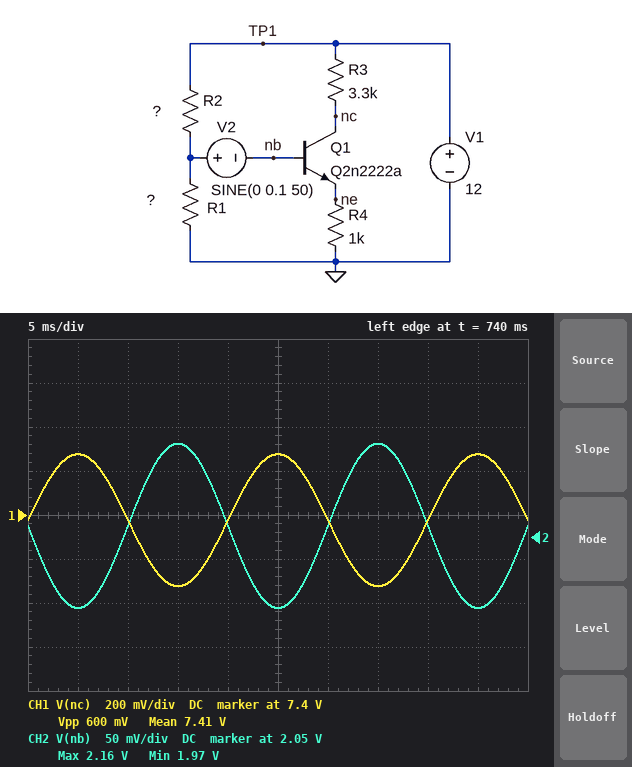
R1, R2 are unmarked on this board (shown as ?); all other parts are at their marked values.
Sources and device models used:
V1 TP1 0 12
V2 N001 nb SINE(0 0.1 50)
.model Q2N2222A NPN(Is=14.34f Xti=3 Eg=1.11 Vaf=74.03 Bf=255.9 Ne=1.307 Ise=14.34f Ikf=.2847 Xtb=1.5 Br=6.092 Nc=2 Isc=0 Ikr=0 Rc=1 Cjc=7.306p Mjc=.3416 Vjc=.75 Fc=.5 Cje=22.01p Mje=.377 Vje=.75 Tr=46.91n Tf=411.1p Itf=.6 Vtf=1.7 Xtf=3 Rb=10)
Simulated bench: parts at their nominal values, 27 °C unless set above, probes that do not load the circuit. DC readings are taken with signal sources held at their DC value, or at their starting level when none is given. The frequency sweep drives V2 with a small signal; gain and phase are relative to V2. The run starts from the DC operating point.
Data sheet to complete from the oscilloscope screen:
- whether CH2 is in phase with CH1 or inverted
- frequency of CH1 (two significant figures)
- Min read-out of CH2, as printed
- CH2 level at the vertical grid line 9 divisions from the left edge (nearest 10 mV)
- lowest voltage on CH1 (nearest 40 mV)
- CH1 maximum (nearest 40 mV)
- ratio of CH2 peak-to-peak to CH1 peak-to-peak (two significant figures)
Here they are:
inverted
50 Hz
1.97 V
1.97 V
7.08 V
7.68 V
0.31
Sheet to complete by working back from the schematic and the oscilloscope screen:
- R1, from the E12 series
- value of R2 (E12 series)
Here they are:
15 kΩ
68 kΩ
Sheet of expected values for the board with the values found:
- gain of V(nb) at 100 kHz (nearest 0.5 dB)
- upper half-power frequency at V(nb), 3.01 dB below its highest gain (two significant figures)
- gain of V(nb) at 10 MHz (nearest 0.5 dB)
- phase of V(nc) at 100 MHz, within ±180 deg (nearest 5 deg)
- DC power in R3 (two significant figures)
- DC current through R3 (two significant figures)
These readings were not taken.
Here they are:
-0.5 dB
810 kHz
-20.5 dB
-165 deg
6.5 mW
1.4 mA
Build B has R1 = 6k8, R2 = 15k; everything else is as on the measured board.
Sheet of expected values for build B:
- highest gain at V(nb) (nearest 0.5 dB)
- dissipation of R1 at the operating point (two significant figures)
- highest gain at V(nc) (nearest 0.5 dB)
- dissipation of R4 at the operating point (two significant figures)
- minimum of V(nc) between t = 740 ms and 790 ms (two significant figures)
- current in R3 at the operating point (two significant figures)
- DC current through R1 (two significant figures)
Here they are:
-15.0 dB
1.8 mW
-17.0 dB
7.9 mW
2.9 V
2.8 mA
510 µA
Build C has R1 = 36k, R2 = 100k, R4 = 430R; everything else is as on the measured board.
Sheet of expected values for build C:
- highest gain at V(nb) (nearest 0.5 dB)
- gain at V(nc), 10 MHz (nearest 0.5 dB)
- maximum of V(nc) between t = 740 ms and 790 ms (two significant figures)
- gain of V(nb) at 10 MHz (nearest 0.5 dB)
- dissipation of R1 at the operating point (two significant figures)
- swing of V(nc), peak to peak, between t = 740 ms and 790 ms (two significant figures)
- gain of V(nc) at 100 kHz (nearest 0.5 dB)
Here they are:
-33.5 dB
-37.0 dB
1.5 V
-36.5 dB
120 µW
4.5 mV
-33.0 dB
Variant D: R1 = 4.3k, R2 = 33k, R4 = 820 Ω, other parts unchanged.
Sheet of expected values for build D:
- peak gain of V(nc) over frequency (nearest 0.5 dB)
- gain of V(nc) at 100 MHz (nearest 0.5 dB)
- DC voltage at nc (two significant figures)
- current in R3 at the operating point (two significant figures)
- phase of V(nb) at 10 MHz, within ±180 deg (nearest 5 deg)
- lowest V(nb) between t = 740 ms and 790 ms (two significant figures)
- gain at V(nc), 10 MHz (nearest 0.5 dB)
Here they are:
11.5 dB
-14.5 dB
9.1 V
880 µA
135 deg
1.3 V
-2.0 dB
